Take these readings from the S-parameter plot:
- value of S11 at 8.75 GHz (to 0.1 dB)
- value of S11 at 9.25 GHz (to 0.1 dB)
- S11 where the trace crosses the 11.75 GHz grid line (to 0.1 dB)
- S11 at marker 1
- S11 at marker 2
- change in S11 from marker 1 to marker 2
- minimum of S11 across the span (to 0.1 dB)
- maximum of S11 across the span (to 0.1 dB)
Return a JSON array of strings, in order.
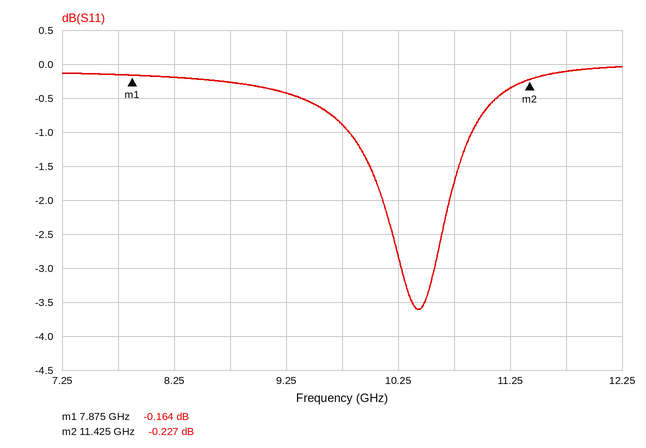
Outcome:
["-0.3 dB", "-0.4 dB", "-0.1 dB", "-0.164 dB", "-0.227 dB", "-0.063 dB", "-3.6 dB", "0.0 dB"]
